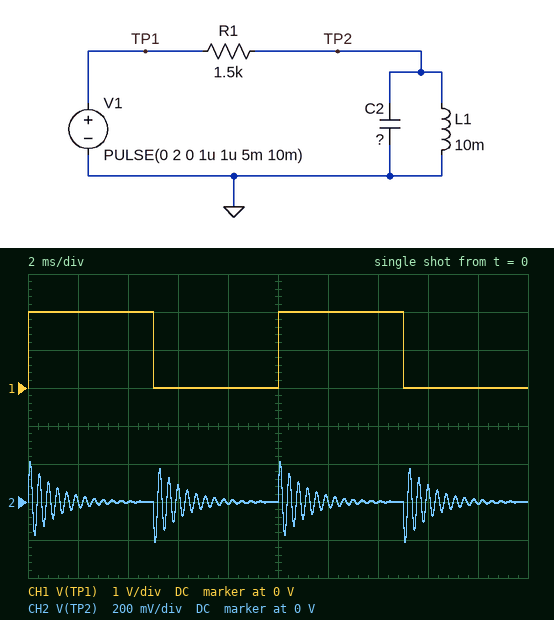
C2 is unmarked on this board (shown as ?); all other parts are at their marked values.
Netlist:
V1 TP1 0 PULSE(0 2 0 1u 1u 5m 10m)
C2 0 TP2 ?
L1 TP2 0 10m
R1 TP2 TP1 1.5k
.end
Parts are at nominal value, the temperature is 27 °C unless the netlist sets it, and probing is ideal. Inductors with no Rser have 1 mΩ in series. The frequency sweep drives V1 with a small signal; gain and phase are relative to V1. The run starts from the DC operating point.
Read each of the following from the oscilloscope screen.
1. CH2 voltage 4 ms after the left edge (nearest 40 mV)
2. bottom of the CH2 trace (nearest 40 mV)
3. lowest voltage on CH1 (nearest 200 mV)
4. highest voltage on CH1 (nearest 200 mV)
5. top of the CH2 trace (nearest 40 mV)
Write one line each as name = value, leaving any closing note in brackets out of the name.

CH2 voltage 4 ms after the left edge = 0 V
bottom of the CH2 trace = -200 mV
lowest voltage on CH1 = 0 V
highest voltage on CH1 = 2.0 V
top of the CH2 trace = 200 mV
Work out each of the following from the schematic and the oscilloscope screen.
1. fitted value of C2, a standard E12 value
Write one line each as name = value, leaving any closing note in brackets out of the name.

fitted value of C2, a standard E12 value = 330 nF
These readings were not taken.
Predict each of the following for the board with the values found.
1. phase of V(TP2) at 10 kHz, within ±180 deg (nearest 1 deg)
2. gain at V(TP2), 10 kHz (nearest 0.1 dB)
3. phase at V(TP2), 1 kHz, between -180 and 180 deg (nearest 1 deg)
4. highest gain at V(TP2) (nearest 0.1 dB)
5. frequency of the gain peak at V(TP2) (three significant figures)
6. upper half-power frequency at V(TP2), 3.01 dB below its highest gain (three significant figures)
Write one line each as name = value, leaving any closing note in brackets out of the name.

phase of V(TP2) at 10 kHz, within ±180 deg = -88 deg
gain at V(TP2), 10 kHz = -29.2 dB
phase at V(TP2), 1 kHz, between -180 and 180 deg = 87 deg
highest gain at V(TP2) = 0 dB
frequency of the gain peak at V(TP2) = 2.77 kHz
upper half-power frequency at V(TP2), 3.01 dB below its highest gain = 2.94 kHz
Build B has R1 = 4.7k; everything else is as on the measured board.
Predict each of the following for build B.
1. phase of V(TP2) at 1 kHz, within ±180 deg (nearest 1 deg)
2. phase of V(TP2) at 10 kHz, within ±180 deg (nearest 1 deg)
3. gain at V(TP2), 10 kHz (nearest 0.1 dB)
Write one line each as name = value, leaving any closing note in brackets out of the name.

phase of V(TP2) at 1 kHz, within ±180 deg = 89 deg
phase of V(TP2) at 10 kHz, within ±180 deg = -89 deg
gain at V(TP2), 10 kHz = -39.1 dB
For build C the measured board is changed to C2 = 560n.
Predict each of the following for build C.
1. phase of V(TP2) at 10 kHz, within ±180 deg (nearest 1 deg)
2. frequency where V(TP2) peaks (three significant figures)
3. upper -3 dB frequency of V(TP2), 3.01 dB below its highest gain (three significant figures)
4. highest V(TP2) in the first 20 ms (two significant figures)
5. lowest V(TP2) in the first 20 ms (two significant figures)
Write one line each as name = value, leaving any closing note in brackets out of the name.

phase of V(TP2) at 10 kHz, within ±180 deg = -89 deg
frequency where V(TP2) peaks = 2.13 kHz
upper -3 dB frequency of V(TP2), 3.01 dB below its highest gain = 2.22 kHz
highest V(TP2) in the first 20 ms = 170 mV
lowest V(TP2) in the first 20 ms = -170 mV
